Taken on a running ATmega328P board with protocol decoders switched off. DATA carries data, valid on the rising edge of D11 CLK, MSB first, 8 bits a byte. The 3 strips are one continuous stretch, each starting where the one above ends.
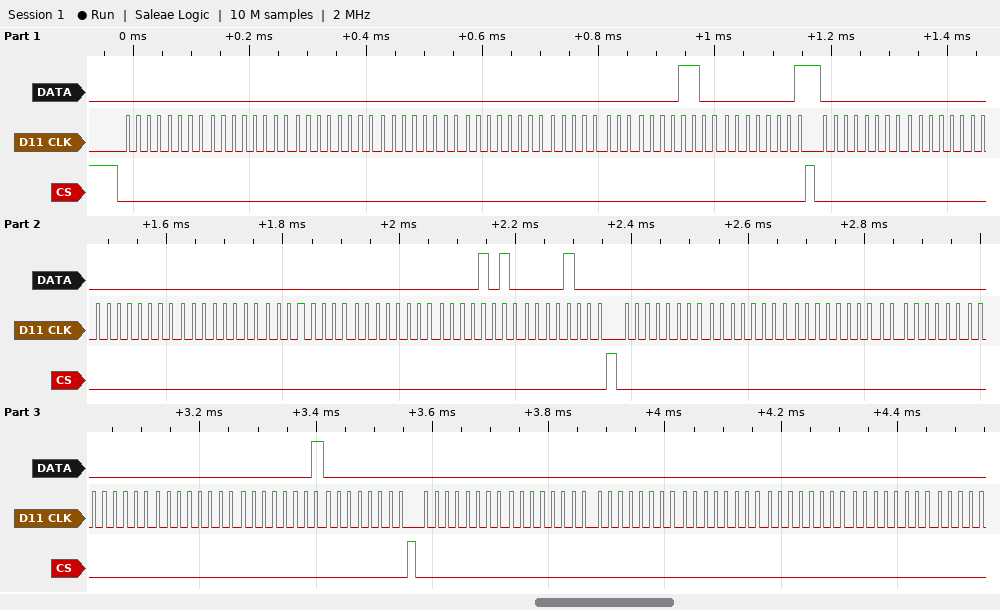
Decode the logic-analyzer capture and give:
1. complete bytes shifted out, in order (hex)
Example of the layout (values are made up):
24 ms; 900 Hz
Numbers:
0x00 0x00 0x00 0x00 0x00 0x00 0x0C 0x01 0x00 0x00 0x00 0x00 0x00 0x00 0x0A 0x08 0x00 0x00 0x00 0x00 0x00 0x00 0x01 0x00 0x00 0x00 0x00 0x00 0x00 0x00
